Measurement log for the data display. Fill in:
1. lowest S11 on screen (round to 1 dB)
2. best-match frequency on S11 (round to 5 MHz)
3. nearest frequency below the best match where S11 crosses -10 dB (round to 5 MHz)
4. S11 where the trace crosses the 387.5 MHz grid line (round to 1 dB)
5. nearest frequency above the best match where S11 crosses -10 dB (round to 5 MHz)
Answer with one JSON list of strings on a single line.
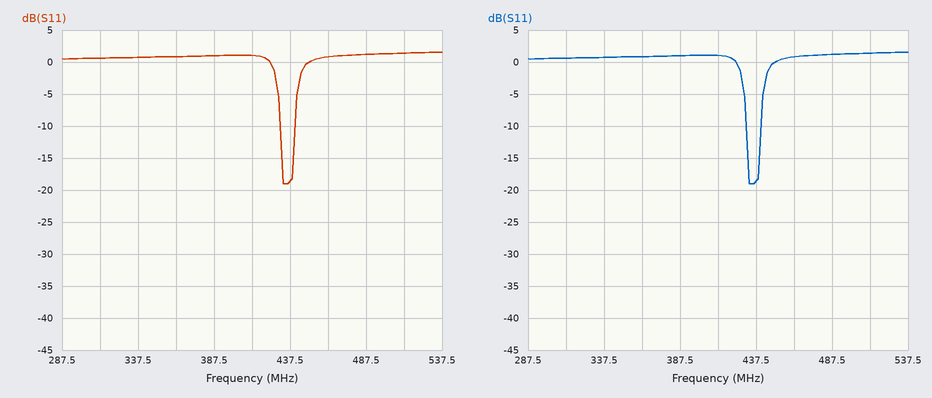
["-19 dB", "435 MHz", "430 MHz", "1 dB", "440 MHz"]
